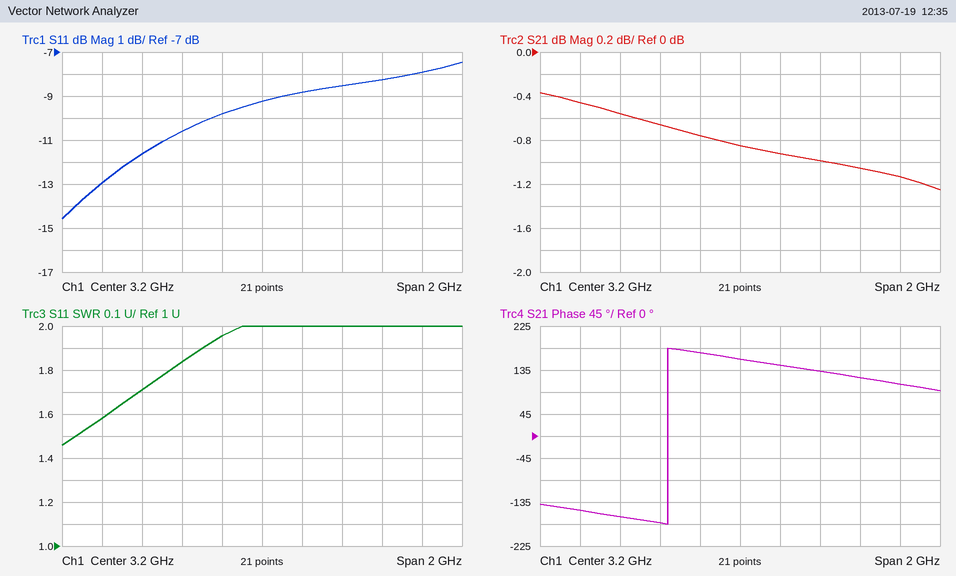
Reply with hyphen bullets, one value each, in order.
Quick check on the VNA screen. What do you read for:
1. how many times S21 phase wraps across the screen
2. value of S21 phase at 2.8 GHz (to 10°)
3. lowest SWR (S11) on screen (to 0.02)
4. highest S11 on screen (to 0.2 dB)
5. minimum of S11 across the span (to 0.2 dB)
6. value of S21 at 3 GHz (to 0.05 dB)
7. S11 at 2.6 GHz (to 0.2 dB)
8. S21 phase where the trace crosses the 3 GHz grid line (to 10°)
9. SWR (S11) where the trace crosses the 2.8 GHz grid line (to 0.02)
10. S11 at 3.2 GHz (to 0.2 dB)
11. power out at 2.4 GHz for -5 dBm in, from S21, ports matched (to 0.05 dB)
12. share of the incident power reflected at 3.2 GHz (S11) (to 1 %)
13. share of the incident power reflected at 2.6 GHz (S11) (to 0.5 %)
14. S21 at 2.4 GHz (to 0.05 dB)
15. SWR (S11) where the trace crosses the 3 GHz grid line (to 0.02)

- 1
- -180°
- 1.46
- -7.4 dB
- -14.6 dB
- -0.75 dB
- -11.6 dB
- 170°
- 1.84
- -9.2 dB
- -5.45 dBm
- 12 %
- 7.0 %
- -0.45 dB
- 1.96
